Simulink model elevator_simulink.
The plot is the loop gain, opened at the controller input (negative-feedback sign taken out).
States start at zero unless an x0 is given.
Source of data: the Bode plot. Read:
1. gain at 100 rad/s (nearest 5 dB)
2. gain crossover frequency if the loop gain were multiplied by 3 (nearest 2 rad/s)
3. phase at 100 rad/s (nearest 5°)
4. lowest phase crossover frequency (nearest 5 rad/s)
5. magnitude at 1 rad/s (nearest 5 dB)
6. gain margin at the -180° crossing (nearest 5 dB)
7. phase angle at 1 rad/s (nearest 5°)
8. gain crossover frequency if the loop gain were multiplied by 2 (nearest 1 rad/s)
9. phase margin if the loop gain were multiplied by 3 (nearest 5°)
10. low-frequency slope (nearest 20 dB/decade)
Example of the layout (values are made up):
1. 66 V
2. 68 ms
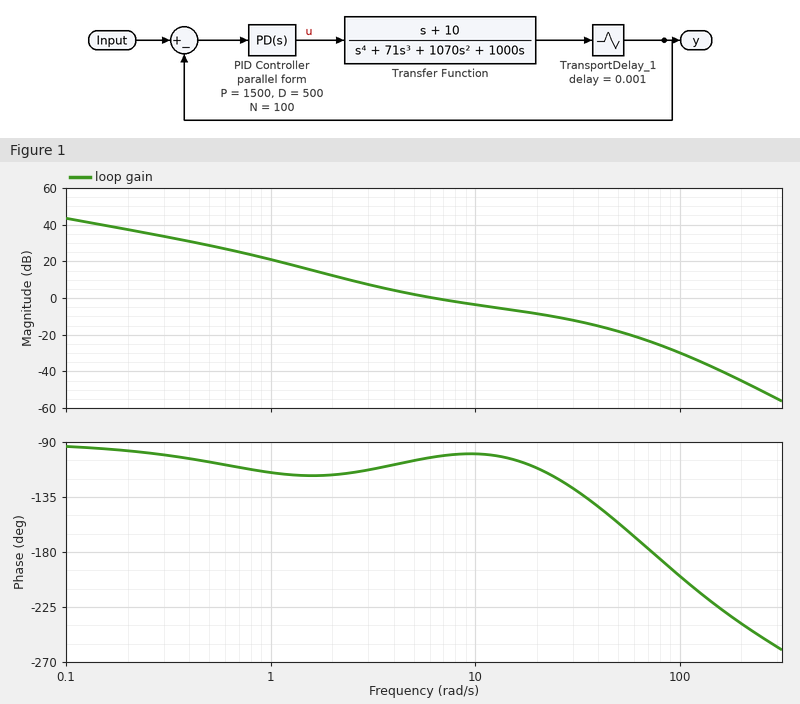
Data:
1. -30 dB
2. 22 rad/s
3. -200°
4. 75 rad/s
5. 20 dB
6. 25 dB
7. -115°
8. 14 rad/s
9. 65°
10. -20 dB/decade
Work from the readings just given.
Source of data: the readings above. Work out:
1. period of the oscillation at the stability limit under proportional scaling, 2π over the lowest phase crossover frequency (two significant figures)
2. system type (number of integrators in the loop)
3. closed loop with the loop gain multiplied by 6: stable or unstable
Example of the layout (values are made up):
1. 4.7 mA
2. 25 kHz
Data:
1. 0.084 s
2. 1
3. stable
